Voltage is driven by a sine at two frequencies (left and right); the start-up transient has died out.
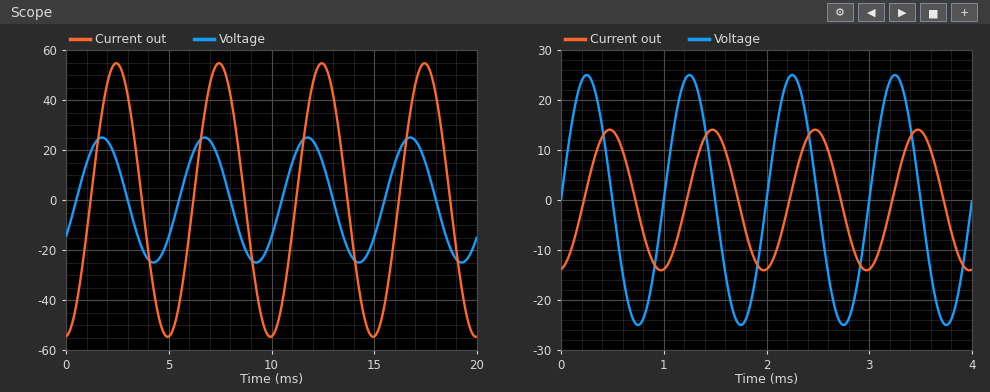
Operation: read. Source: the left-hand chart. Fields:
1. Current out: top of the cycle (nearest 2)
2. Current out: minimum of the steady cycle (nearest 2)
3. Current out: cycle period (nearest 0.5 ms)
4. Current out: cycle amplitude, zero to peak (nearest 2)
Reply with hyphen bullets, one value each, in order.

- 54
- -54
- 5.0 ms
- 54
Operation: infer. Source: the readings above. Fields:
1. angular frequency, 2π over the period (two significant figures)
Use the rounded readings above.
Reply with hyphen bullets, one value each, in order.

- 1.3 rad/ms
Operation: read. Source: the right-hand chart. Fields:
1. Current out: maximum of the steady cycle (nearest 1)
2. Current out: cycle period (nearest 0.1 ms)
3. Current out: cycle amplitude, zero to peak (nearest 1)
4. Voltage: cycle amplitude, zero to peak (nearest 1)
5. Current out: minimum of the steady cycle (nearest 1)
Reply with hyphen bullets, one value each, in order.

- 14
- 1.0 ms
- 14
- 25
- -14
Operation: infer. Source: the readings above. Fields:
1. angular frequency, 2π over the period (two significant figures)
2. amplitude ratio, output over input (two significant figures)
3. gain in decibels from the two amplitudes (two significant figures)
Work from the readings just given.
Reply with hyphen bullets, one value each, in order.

- 6.3 rad/ms
- 0.56
- -5.0 dB
